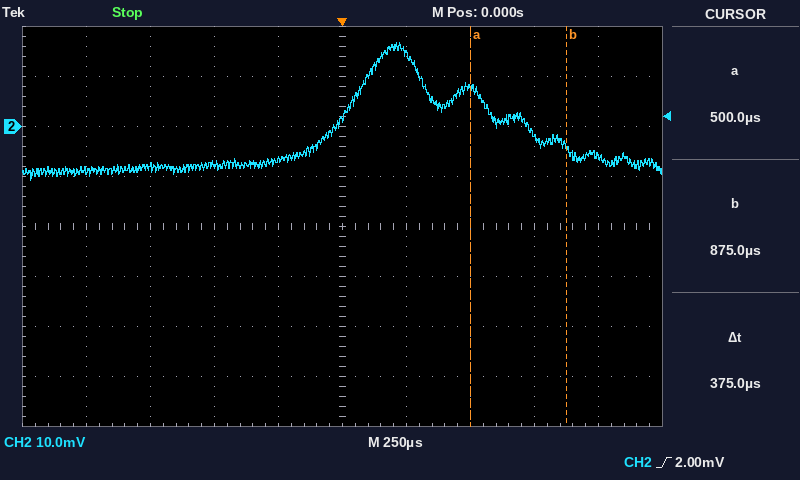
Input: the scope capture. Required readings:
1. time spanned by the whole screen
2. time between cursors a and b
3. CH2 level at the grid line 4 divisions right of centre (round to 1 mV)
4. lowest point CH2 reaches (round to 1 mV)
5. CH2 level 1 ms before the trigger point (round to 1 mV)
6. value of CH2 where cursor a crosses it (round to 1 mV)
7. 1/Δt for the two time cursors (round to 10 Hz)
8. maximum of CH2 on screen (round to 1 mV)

2.5 ms
375 µs
-6 mV
-11 mV
-9 mV
8 mV
2.67 kHz
17 mV
